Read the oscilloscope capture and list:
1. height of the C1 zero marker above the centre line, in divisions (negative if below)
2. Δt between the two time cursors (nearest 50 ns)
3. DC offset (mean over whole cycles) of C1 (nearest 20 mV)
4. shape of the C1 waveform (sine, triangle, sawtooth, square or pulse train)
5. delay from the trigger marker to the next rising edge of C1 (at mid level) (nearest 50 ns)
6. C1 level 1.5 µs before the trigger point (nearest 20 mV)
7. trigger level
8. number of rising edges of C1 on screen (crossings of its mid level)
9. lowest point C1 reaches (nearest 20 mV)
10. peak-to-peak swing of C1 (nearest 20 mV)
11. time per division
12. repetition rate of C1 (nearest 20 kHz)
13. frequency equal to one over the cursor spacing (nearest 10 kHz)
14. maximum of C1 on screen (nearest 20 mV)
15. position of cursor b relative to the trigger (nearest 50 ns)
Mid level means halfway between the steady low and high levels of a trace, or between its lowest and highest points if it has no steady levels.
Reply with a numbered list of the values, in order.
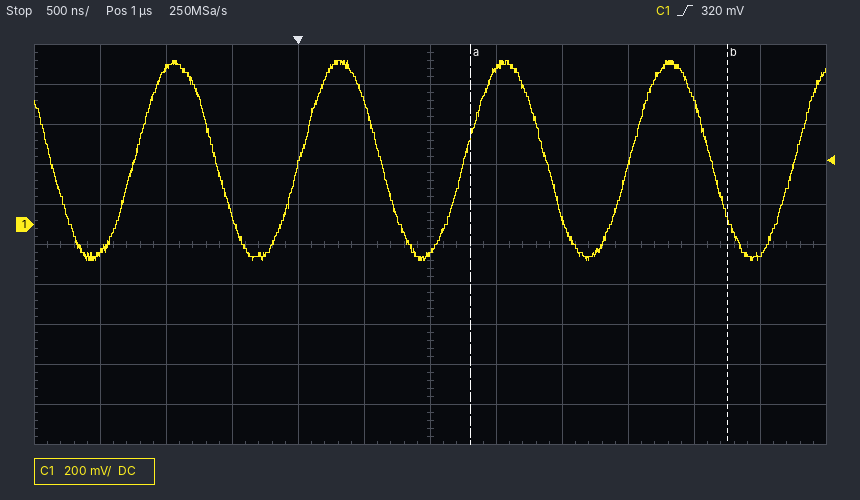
1. +0.5 div
2. 1.95 µs
3. 320 mV
4. sine
5. 1.25 µs
6. -140 mV
7. 320 mV
8. 5
9. -180 mV
10. 1.00 V
11. 500 ns
12. 800 kHz
13. 510 kHz
14. 820 mV
15. +3.25 µs
